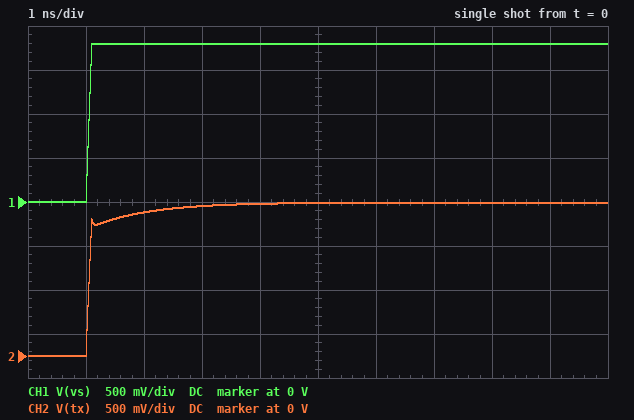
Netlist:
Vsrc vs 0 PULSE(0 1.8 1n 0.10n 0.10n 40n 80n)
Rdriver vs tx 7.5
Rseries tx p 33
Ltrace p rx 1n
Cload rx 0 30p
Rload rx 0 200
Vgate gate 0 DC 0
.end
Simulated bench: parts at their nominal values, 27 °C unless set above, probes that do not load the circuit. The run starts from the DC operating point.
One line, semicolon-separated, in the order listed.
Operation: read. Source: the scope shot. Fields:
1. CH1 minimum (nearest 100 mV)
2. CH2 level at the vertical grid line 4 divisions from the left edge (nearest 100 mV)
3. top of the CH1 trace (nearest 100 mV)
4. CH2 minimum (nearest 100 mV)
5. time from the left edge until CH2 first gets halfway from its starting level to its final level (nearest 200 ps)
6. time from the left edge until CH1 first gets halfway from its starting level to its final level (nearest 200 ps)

0 V; 1.7 V; 1.8 V; 0 V; 1.0 ns; 1.0 ns
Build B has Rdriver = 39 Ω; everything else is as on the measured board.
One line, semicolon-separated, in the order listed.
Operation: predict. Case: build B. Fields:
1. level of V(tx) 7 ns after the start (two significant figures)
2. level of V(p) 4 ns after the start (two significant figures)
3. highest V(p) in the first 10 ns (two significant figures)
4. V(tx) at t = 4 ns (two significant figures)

1.5 V; 1.1 V; 1.3 V; 1.4 V
